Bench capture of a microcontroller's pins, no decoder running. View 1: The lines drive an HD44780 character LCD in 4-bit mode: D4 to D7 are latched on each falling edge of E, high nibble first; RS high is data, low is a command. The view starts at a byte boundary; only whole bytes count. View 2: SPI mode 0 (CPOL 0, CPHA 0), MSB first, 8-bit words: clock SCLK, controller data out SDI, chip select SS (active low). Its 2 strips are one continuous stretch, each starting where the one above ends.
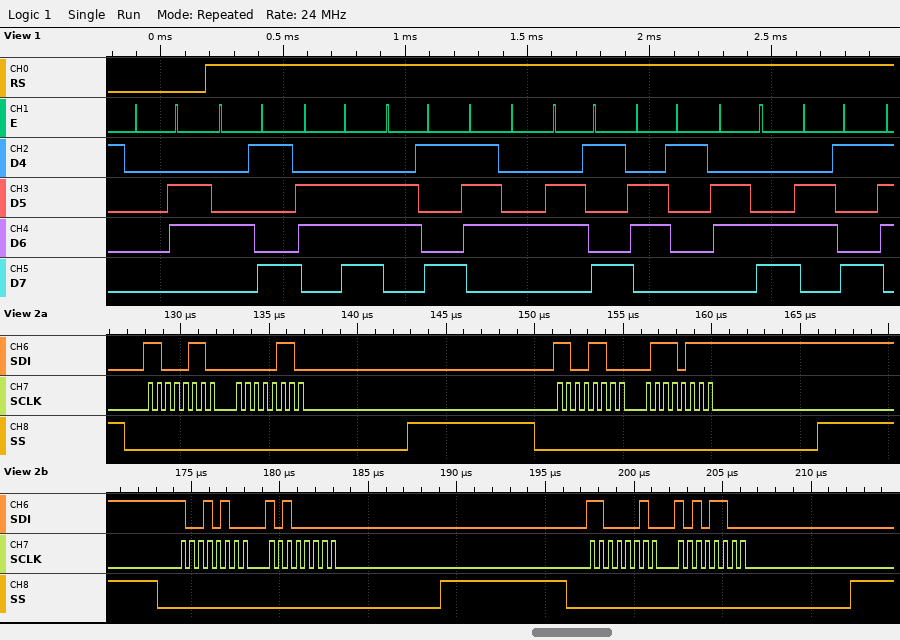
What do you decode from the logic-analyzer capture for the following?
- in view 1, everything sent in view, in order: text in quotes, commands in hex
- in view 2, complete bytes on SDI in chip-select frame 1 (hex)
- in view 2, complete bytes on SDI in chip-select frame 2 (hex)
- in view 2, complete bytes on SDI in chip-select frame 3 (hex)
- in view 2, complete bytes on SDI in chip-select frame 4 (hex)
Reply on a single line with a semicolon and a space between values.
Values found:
0x06 "Initiali"; 0xC6 0x06; 0xCC 0x77; 0x94 0xA0; 0xC2 0xAC
